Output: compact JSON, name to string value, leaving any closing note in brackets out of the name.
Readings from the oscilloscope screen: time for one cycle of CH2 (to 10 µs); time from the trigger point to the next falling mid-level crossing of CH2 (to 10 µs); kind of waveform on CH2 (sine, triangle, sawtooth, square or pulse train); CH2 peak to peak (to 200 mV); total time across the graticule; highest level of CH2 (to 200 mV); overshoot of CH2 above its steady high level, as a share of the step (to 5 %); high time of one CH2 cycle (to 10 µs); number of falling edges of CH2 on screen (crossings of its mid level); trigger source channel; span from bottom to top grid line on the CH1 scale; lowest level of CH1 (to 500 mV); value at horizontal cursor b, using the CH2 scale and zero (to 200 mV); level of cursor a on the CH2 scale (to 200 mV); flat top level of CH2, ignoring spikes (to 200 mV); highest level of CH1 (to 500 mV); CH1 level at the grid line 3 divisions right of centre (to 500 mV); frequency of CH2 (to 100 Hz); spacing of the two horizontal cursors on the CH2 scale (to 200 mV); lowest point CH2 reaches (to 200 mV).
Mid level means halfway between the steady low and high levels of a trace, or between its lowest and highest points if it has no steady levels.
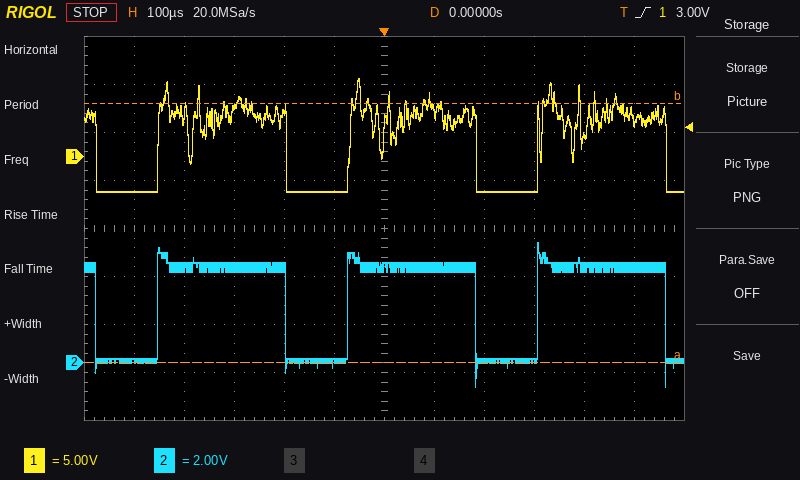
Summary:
{"time for one cycle of CH2": "380 µs", "time from the trigger point to the next falling mid-level crossing of CH2": "180 µs", "kind of waveform on CH2": "pulse train", "CH2 peak to peak": "6.0 V", "total time across the graticule": "1.2 ms", "highest level of CH2": "5.0 V", "overshoot of CH2 above its steady high level, as a share of the step": "25 %", "high time of one CH2 cycle": "260 µs", "number of falling edges of CH2 on screen": "4", "trigger source channel": "CH1", "span from bottom to top grid line on the CH1 scale": "40 V", "lowest level of CH1": "-3.5 V", "value at horizontal cursor b, using the CH2 scale and zero": "10.8 V", "level of cursor a on the CH2 scale": "0.0 V", "flat top level of CH2, ignoring spikes": "4.0 V", "highest level of CH1": "8.0 V", "CH1 level at the grid line 3 divisions right of centre": "-3.5 V", "frequency of CH2": "2.6 kHz", "spacing of the two horizontal cursors on the CH2 scale": "10.8 V", "lowest point CH2 reaches": "-1.0 V"}
